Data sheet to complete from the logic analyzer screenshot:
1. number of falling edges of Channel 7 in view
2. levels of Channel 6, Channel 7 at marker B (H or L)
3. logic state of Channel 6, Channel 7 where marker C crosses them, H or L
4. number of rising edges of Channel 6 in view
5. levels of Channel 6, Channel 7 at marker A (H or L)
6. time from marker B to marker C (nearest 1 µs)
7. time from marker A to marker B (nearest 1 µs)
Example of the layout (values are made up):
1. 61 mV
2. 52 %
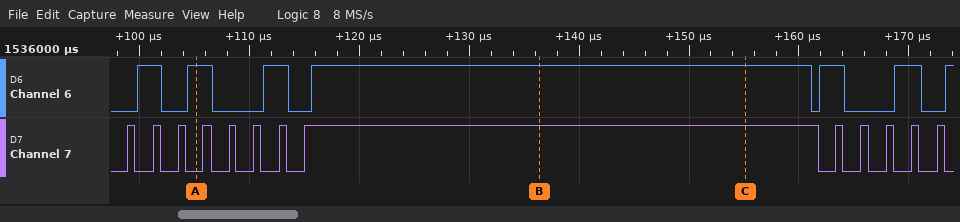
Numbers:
1. 13
2. Channel 6=H, Channel 7=H
3. Channel 6=H, Channel 7=H
4. 7
5. Channel 6=H, Channel 7=L
6. 19 µs
7. 31 µs
